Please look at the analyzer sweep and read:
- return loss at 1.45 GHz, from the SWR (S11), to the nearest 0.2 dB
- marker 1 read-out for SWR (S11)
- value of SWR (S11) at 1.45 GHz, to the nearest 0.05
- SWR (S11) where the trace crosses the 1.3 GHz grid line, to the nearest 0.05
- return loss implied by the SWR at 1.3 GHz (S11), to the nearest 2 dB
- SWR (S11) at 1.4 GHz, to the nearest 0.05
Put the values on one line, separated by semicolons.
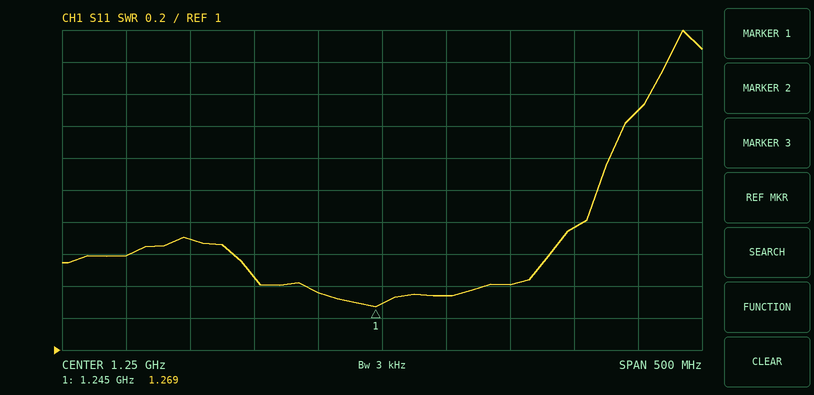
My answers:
7.4 dB; 1.269; 2.50; 1.35; 16 dB; 1.75
